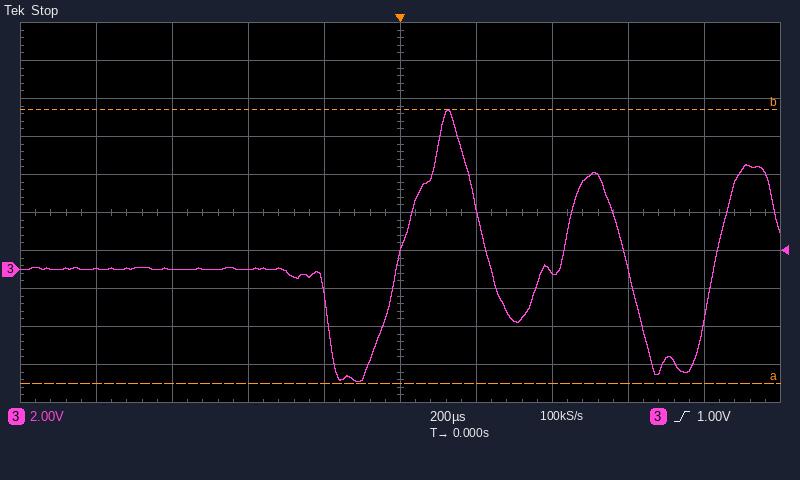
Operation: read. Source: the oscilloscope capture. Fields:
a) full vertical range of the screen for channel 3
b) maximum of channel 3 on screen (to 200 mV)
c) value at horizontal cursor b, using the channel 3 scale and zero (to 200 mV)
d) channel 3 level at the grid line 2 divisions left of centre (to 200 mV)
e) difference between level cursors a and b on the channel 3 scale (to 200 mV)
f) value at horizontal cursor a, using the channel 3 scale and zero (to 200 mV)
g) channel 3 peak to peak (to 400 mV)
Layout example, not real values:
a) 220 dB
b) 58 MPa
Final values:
a) 20 V
b) 8.4 V
c) 8.4 V
d) 0.0 V
e) 14.4 V
f) -6.0 V
g) 14.4 V
